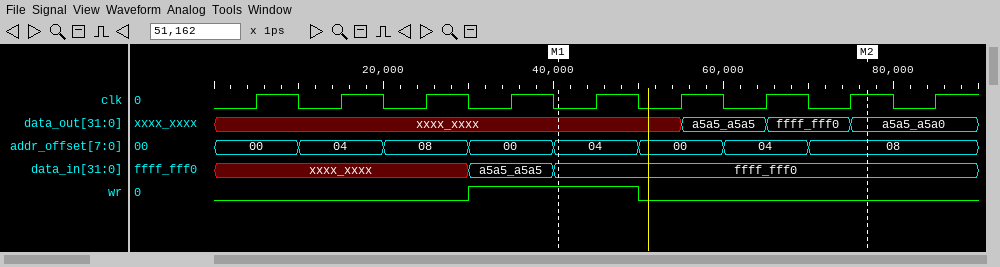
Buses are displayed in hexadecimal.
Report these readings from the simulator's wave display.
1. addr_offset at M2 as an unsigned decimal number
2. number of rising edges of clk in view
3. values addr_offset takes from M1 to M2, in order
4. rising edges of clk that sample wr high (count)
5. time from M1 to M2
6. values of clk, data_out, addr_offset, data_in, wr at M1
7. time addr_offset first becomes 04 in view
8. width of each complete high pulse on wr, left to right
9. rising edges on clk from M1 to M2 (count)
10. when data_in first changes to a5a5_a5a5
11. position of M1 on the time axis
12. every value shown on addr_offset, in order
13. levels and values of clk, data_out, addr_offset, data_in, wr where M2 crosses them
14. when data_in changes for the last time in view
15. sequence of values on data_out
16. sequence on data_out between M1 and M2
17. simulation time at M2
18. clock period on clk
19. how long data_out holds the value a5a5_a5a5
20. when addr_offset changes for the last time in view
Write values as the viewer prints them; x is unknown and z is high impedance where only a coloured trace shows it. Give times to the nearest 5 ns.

8
9
04, 00, 04, 08
2
35 ns
clk=0, data_out=xxxx_xxxx, addr_offset=04, data_in=ffff_fff0, wr=1
10 ns
20 ns
4
30 ns
40 ns
00, 04, 08, 00, 04, 00, 04, 08
clk=1, data_out=a5a5_a5a0, addr_offset=08, data_in=ffff_fff0, wr=0
40 ns
xxxx_xxxx, a5a5_a5a5, ffff_fff0, a5a5_a5a0
xxxx_xxxx, a5a5_a5a5, ffff_fff0, a5a5_a5a0
75 ns
10 ns
10 ns
70 ns
